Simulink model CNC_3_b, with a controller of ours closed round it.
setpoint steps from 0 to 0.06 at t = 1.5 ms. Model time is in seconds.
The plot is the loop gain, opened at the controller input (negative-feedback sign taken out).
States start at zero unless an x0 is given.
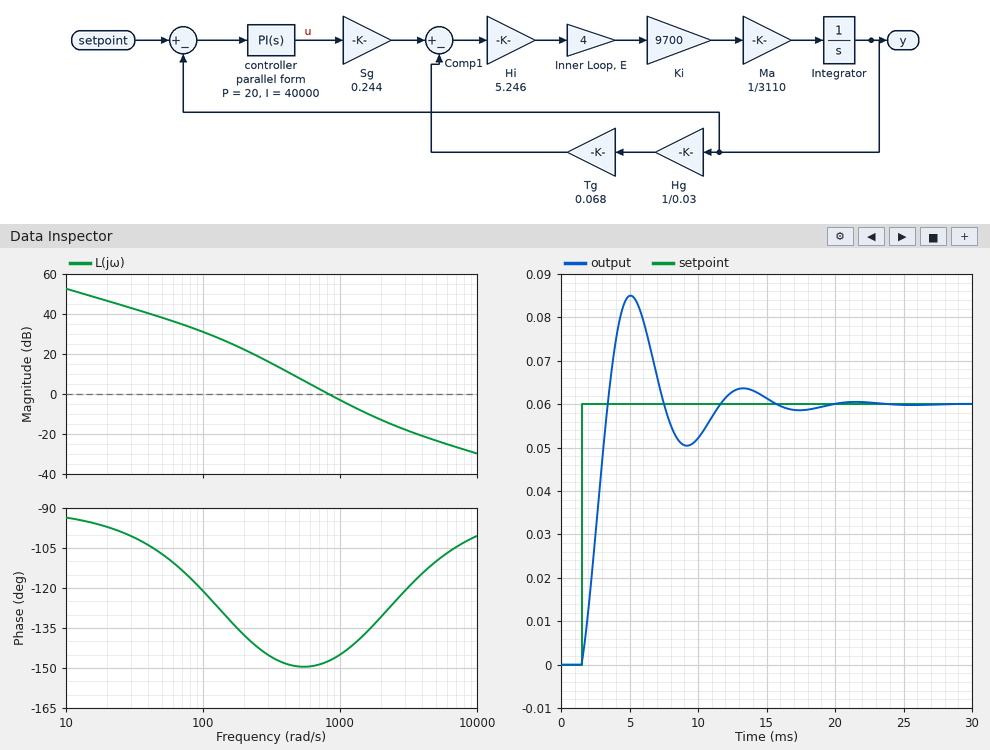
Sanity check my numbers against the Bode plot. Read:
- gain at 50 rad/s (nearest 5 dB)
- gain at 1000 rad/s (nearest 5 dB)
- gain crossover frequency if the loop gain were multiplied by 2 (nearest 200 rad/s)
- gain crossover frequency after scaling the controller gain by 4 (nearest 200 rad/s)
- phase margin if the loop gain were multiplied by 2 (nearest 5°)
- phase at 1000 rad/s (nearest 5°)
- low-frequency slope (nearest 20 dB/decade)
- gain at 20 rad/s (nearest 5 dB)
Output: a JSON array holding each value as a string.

["40 dB", "-5 dB", "1200 rad/s", "1800 rad/s", "40°", "-145°", "-20 dB/decade", "45 dB"]
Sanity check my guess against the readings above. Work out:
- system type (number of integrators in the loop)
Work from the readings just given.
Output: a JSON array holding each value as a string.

["1"]
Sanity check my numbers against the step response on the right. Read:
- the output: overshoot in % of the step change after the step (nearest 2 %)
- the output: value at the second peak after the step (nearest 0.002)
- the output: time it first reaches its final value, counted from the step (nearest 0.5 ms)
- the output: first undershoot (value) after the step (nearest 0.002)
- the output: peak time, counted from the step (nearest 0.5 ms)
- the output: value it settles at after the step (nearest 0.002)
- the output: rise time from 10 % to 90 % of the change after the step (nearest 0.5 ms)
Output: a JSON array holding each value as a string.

["42 %", "0.064", "2.0 ms", "0.050", "3.5 ms", "0.060", "1.5 ms"]
